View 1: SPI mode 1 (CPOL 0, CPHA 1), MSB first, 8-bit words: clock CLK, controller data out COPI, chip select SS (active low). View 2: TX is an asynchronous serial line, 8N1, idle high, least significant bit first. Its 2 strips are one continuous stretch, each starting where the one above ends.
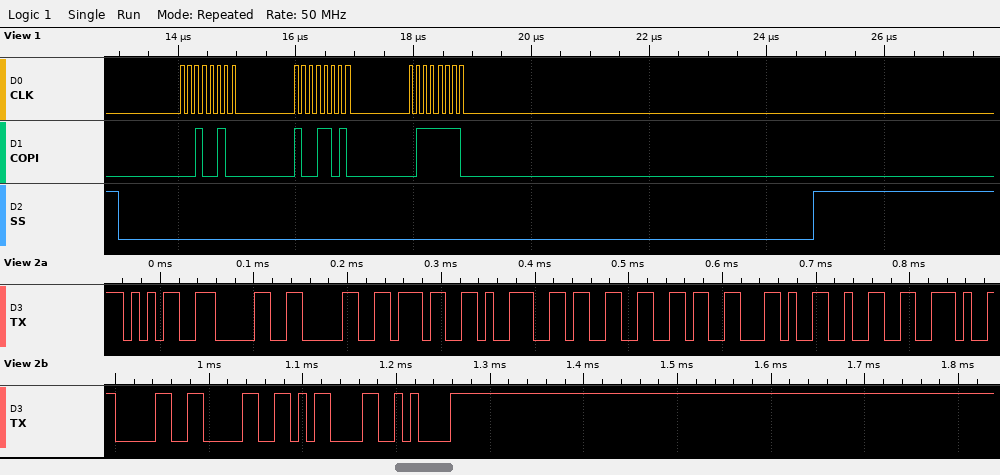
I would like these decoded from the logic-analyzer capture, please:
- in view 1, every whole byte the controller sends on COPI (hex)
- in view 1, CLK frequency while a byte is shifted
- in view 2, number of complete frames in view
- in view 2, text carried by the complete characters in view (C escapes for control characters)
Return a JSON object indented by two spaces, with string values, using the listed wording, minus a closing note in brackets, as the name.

{
  "in view 1, every whole byte the controller sends on COPI": "0x24 0x9A 0x7E",
  "in view 1, CLK frequency while a byte is shifted": "8 MHz",
  "in view 2, number of complete frames in view": "14",
  "in view 2, text carried by the complete characters in view": "\"5007936,2.00\\r\\n\""
}
